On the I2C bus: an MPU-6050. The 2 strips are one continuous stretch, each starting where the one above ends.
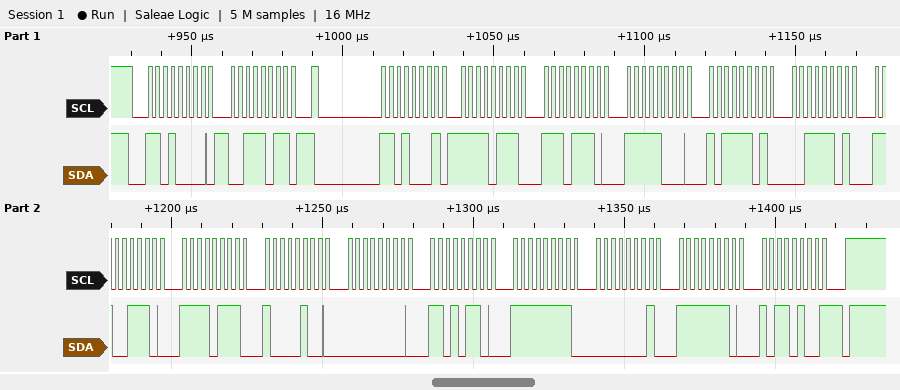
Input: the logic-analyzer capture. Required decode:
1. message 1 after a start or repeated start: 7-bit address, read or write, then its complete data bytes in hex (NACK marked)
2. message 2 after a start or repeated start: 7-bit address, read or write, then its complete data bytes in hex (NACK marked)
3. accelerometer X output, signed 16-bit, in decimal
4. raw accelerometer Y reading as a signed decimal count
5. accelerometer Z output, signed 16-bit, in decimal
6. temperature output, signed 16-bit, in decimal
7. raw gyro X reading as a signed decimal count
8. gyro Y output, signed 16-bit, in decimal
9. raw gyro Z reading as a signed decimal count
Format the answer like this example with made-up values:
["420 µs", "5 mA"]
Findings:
["0x68 write: 3B", "0x68 read: F7 EE F8 BD 3D CE F7 84 00 D6 FF 01 FE B4 NACK", "-2066", "-1859", "15822", "-2172", "214", "-255", "-332"]
